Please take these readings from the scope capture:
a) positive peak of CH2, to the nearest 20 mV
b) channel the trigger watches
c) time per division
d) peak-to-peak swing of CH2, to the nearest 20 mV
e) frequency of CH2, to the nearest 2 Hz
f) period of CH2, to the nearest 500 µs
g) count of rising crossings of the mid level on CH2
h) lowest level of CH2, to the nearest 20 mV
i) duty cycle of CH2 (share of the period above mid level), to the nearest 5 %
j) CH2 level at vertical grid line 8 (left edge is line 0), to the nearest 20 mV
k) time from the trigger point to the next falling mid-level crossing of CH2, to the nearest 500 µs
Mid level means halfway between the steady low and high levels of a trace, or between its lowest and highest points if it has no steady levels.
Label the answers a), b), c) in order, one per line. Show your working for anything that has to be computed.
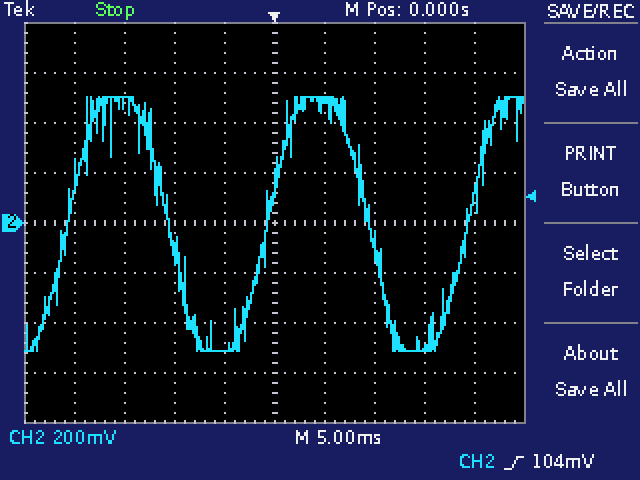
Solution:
a) 500 mV
b) CH2
c) 5 ms
d) 500 mV − (-520 mV) = 1.02 V
e) 1 / 20.0 ms ≈ 50 Hz
f) 20.0 ms
g) 3
h) -520 mV
i) 50 %
j) -500 mV
k) 9.5 ms
